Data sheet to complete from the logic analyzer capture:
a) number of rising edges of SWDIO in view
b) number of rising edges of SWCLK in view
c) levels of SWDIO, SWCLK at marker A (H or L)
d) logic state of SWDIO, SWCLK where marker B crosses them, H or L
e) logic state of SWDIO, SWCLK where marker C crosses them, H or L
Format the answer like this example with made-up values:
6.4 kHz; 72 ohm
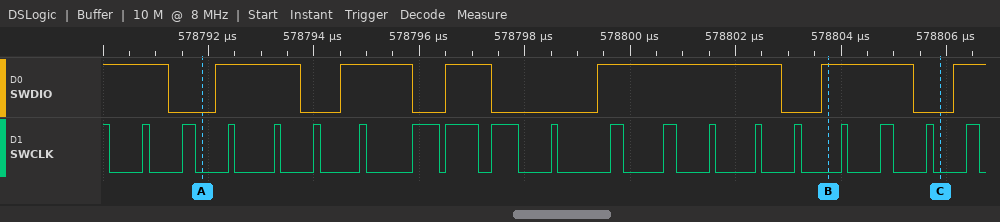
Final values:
6; 19; SWDIO=L, SWCLK=L; SWDIO=H, SWCLK=L; SWDIO=L, SWCLK=L
